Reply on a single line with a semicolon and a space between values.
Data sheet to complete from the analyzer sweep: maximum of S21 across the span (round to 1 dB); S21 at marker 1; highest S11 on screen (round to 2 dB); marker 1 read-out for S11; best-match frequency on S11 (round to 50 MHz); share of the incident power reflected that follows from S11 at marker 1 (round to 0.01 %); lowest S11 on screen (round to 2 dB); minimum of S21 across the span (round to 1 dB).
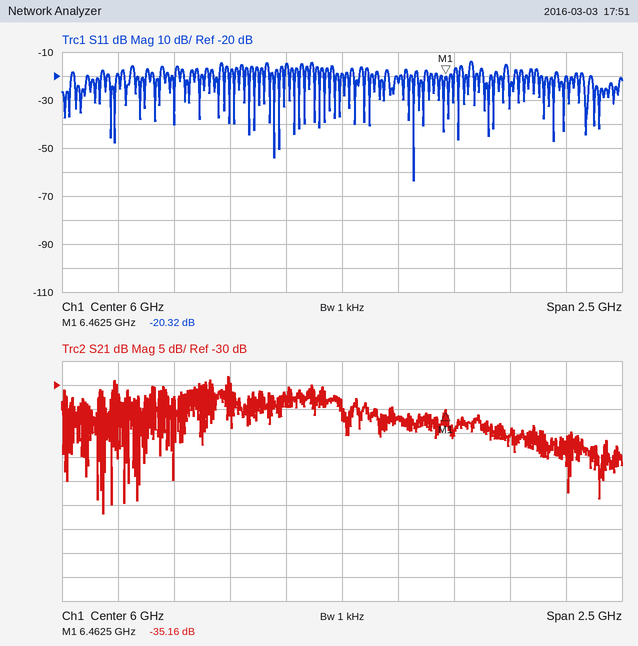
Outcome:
-28 dB; -35.16 dB; -14 dB; -20.32 dB; 6.30 GHz; 0.93 %; -64 dB; -57 dB
